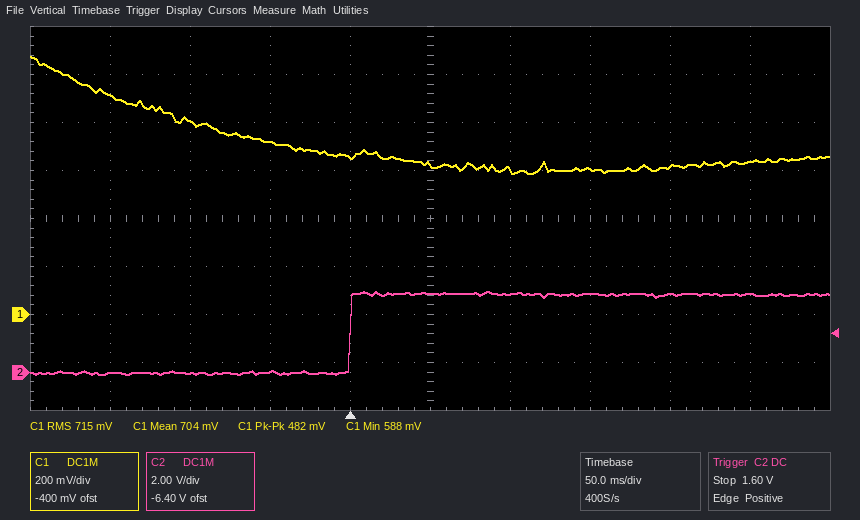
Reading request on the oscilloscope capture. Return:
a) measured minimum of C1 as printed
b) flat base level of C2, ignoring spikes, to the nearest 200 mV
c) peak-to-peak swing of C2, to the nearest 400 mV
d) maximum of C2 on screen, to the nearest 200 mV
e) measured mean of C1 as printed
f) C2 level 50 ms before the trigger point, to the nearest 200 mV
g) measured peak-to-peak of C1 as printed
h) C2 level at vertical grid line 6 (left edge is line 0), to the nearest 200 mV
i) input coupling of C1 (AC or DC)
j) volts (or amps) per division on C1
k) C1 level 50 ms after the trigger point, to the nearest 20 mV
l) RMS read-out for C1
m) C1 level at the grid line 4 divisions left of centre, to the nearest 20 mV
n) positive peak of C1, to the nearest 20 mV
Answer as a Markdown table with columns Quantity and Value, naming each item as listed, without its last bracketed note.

| Quantity | Value |
|---|---|
| measured minimum of C1 as printed | 588 mV |
| flat base level of C2, ignoring spikes, to the nearest 200 mV | 0.0 V |
| peak-to-peak swing of C2, to the nearest 400 mV | 3.6 V |
| maximum of C2 on screen, to the nearest 200 mV | 3.4 V |
| measured mean of C1 as printed | 704 mV |
| C2 level 50 ms before the trigger point, to the nearest 200 mV | 0.0 V |
| measured peak-to-peak of C1 as printed | 482 mV |
| C2 level at vertical grid line 6 (left edge is line 0), to the nearest 200 mV | 3.2 V |
| input coupling of C1 | DC |
| volts (or amps) per division on C1 | 200 mV |
| C1 level 50 ms after the trigger point, to the nearest 20 mV | 620 mV |
| RMS read-out for C1 | 715 mV |
| C1 level at the grid line 4 divisions left of centre, to the nearest 20 mV | 920 mV |
| positive peak of C1, to the nearest 20 mV | 1.08 V |
